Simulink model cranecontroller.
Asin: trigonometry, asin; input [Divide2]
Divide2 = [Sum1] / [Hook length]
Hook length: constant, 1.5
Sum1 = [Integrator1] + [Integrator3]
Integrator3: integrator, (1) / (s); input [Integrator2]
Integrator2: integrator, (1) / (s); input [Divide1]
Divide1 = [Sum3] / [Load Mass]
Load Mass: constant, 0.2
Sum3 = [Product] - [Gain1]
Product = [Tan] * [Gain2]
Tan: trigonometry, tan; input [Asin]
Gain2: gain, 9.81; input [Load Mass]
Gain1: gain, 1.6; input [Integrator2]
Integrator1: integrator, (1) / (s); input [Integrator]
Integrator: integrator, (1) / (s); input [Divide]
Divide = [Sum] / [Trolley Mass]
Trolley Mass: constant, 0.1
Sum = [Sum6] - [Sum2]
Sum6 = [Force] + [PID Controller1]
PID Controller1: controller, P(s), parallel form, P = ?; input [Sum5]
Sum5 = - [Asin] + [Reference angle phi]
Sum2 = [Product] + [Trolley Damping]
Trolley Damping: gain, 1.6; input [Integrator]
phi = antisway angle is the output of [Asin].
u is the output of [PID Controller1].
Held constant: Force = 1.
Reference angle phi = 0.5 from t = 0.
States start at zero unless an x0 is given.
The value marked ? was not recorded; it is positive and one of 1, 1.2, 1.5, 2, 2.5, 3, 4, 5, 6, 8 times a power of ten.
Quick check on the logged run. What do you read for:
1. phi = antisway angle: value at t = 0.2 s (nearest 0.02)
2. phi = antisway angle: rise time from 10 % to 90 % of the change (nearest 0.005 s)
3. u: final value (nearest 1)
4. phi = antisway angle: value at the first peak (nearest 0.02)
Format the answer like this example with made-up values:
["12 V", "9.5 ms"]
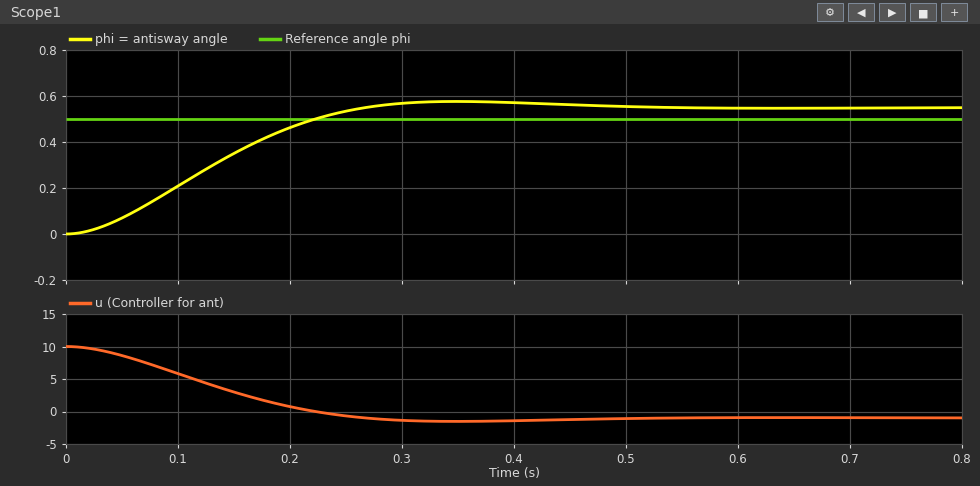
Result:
["0.46", "0.175 s", "-1", "0.58"]
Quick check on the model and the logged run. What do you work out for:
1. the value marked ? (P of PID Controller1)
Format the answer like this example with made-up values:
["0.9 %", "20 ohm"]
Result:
["20"]
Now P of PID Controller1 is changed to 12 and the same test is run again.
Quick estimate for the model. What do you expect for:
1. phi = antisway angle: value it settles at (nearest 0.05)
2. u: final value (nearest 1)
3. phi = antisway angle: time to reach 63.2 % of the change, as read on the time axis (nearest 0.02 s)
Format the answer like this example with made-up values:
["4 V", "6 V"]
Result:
["0.60", "-1", "0.22 s"]
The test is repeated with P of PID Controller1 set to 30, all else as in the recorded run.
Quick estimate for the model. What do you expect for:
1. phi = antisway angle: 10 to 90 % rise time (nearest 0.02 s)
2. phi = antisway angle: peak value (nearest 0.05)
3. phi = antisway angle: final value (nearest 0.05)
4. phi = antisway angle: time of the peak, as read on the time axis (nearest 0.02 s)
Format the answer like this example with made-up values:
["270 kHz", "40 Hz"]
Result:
["0.12 s", "0.60", "0.55", "0.26 s"]
